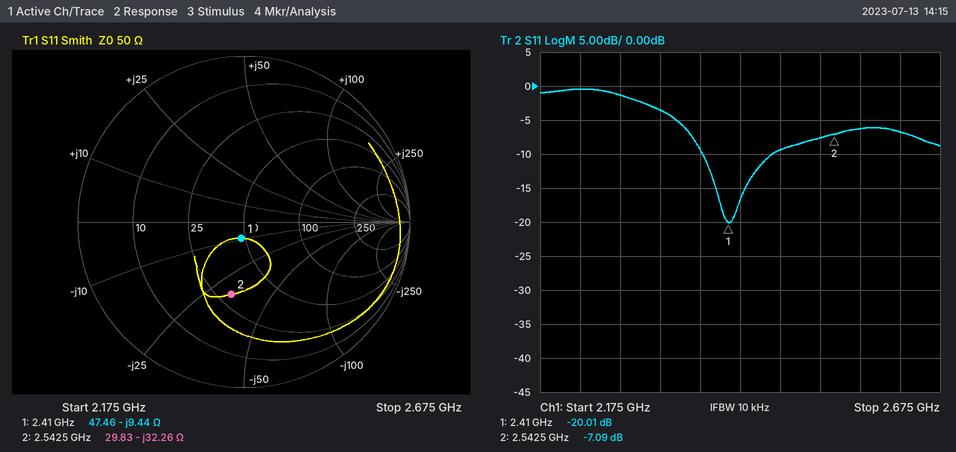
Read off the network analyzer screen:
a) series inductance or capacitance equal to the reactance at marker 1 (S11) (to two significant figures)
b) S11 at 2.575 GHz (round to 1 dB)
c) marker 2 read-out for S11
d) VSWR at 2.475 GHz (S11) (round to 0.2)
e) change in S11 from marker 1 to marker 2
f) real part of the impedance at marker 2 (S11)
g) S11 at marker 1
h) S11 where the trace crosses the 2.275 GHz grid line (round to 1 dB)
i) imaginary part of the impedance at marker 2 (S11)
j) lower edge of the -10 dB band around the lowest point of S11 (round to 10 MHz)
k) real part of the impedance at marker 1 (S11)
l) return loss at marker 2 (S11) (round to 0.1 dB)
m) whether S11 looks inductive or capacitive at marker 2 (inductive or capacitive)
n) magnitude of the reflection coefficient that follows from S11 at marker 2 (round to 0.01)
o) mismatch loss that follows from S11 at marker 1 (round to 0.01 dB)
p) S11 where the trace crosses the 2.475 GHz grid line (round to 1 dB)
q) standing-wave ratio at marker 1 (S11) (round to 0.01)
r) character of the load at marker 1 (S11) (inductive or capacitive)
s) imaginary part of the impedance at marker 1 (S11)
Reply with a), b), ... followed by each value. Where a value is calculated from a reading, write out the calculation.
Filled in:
a) C = 1/(2π × 2.41 GHz × 9.44 Ω) ≈ 7.0 pF
b) -6 dB
c) -7.09 dB
d) |Γ| = 10^(-9/20) = 0.3548; VSWR = (1 + 0.3548)/(1 − 0.3548) ≈ 2.10, so 2.0 to the nearest 0.2
e) -7.09 − (-20.01) = 12.92 dB
f) 29.83 Ω
g) -20.01 dB
h) -1 dB
i) -32.26 Ω
j) 2.38 GHz
k) 47.46 Ω
l) 7.1 dB
m) capacitive
n) 10^(-7.09/20) ≈ 0.44
o) −10 log10(1 − 10^(-20.01/10)) ≈ 0.04 dB
p) -9 dB
q) 1.22
r) capacitive
s) -9.44 Ω
